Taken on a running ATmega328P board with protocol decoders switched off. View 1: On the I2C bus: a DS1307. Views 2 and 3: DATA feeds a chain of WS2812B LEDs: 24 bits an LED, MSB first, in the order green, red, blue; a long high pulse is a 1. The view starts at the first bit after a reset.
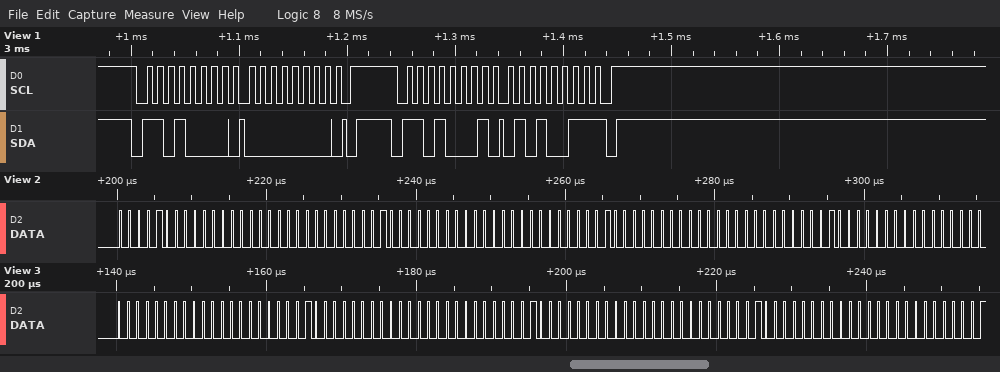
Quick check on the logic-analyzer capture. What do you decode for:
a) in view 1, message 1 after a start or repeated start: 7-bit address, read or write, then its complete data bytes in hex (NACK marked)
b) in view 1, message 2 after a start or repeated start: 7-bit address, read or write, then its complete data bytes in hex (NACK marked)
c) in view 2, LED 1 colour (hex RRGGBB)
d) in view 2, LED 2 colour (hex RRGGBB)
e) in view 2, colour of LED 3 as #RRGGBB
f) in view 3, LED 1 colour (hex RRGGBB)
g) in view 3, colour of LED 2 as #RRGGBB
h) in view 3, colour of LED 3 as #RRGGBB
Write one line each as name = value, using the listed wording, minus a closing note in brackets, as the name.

in view 1, message 1 after a start or repeated start: 7-bit address, read or write, then its complete data bytes in hex = 0x68 write: 00
in view 1, message 2 after a start or repeated start: 7-bit address, read or write, then its complete data bytes in hex = 0x68 read: 53 NACK
in view 2, LED 1 colour = #000800
in view 2, LED 2 colour = #000800
in view 2, colour of LED 3 as #RRGGBB = #000800
in view 3, LED 1 colour = #000008
in view 3, colour of LED 2 as #RRGGBB = #000008
in view 3, colour of LED 3 as #RRGGBB = #000008
